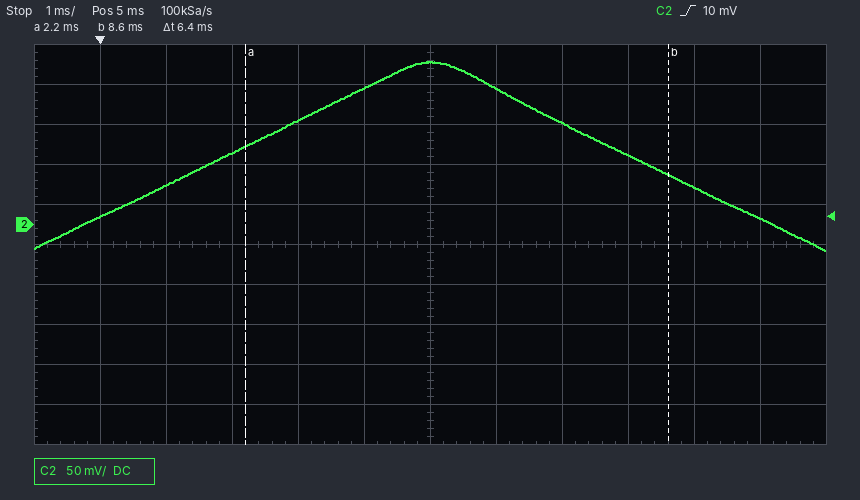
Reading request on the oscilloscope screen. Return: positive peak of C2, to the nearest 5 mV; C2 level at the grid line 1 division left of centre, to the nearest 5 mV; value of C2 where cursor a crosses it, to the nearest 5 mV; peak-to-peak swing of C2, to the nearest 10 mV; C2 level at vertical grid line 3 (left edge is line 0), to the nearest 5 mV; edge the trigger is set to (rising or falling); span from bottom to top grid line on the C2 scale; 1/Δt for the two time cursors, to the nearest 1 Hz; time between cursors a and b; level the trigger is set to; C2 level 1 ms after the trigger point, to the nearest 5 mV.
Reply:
205 mV
170 mV
100 mV
240 mV
90 mV
rising
500 mV
156 Hz
6.4 ms
10 mV
50 mV
